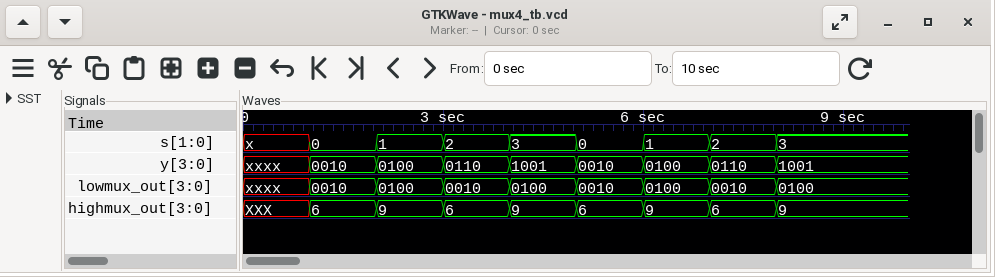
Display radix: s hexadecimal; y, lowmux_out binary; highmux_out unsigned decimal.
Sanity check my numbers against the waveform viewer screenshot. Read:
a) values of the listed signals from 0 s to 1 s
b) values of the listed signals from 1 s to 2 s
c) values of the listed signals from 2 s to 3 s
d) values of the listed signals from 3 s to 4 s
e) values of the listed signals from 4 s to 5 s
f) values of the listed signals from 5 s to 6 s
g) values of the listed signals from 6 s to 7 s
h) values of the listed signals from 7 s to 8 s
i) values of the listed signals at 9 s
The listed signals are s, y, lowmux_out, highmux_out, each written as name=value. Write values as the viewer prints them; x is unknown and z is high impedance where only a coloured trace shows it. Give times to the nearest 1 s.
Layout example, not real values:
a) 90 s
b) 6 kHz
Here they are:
a) s=x, y=xxxx, lowmux_out=xxxx, highmux_out=XXX
b) s=0, y=0010, lowmux_out=0010, highmux_out=6
c) s=1, y=0100, lowmux_out=0100, highmux_out=9
d) s=2, y=0110, lowmux_out=0010, highmux_out=6
e) s=3, y=1001, lowmux_out=0100, highmux_out=9
f) s=0, y=0010, lowmux_out=0010, highmux_out=6
g) s=1, y=0100, lowmux_out=0100, highmux_out=9
h) s=2, y=0110, lowmux_out=0010, highmux_out=6
i) s=3, y=1001, lowmux_out=0100, highmux_out=9
